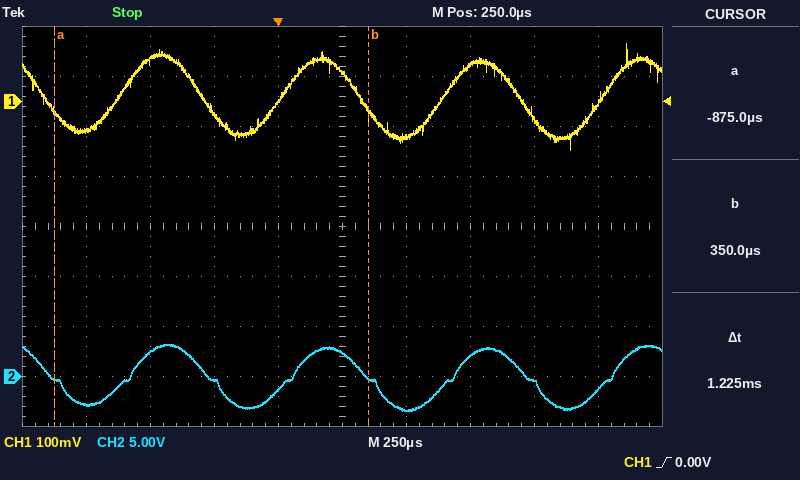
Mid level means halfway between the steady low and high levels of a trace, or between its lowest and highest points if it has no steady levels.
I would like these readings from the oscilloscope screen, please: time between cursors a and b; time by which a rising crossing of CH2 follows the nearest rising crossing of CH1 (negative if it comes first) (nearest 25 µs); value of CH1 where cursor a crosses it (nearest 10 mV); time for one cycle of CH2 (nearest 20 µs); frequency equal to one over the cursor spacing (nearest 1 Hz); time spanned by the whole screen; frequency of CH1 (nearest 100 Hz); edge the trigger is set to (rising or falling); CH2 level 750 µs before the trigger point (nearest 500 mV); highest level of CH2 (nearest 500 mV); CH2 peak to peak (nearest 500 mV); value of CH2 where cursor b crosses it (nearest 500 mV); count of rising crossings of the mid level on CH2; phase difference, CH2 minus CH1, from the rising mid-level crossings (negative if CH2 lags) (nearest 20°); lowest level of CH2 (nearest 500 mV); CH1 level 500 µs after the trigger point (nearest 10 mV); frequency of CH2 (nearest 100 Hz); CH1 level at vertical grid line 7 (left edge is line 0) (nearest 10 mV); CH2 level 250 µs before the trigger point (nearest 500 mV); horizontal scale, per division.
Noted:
1.225 ms
+50 µs
-20 mV
620 µs
816 Hz
2.5 ms
1.6 kHz
rising
-3.0 V
3.0 V
6.5 V
0.0 V
4
-20°
-3.5 V
-70 mV
1.6 kHz
70 mV
-500 mV
250 µs
